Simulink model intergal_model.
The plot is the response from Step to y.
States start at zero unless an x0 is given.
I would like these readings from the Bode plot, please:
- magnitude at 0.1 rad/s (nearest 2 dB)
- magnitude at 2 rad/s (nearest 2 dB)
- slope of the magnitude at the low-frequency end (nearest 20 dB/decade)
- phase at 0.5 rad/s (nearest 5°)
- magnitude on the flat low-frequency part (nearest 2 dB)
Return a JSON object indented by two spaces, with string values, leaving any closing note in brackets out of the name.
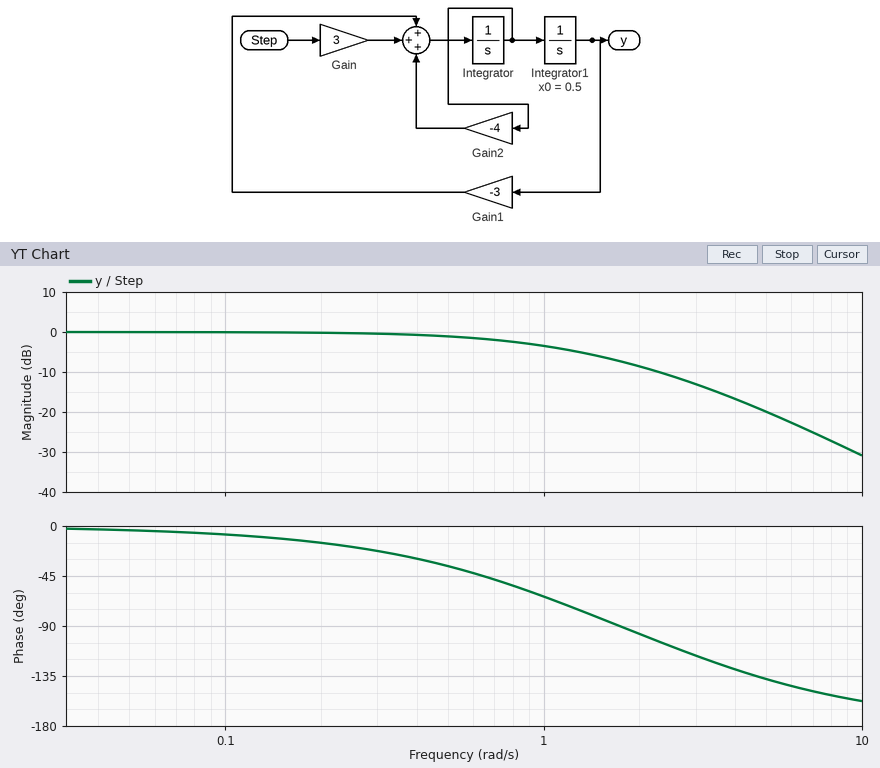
{
  "magnitude at 0.1 rad/s": "0 dB",
  "magnitude at 2 rad/s": "-8 dB",
  "slope of the magnitude at the low-frequency end": "0 dB/decade",
  "phase at 0.5 rad/s": "-35°",
  "magnitude on the flat low-frequency part": "0 dB"
}
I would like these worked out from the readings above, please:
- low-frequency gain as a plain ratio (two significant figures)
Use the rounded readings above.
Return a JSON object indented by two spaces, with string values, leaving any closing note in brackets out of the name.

{
  "low-frequency gain as a plain ratio": "1.0"
}
